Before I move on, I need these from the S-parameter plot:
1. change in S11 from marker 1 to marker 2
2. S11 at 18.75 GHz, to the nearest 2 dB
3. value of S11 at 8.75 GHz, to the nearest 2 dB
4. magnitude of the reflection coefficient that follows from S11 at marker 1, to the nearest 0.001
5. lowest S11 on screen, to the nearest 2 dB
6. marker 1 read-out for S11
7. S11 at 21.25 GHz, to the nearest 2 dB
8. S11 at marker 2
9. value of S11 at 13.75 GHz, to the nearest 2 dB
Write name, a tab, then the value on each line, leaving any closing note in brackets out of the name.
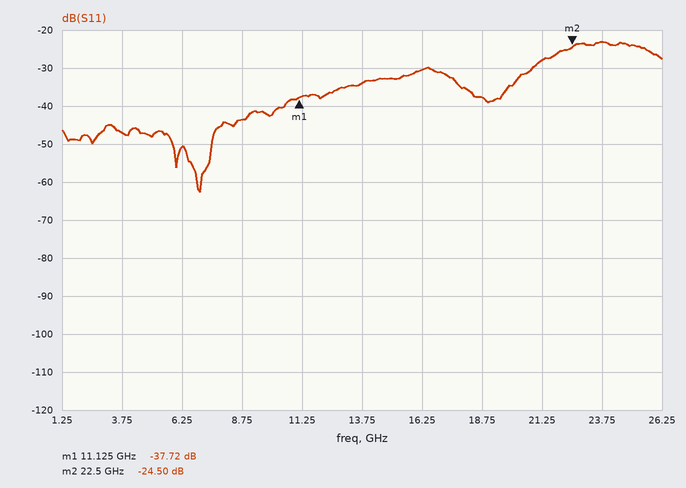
change in S11 from marker 1 to marker 2	13.22 dB
S11 at 18.75 GHz, to the nearest 2 dB	-38 dB
value of S11 at 8.75 GHz, to the nearest 2 dB	-44 dB
magnitude of the reflection coefficient that follows from S11 at marker 1, to the nearest 0.001	0.013
lowest S11 on screen, to the nearest 2 dB	-62 dB
marker 1 read-out for S11	-37.72 dB
S11 at 21.25 GHz, to the nearest 2 dB	-28 dB
S11 at marker 2	-24.50 dB
value of S11 at 13.75 GHz, to the nearest 2 dB	-34 dB
